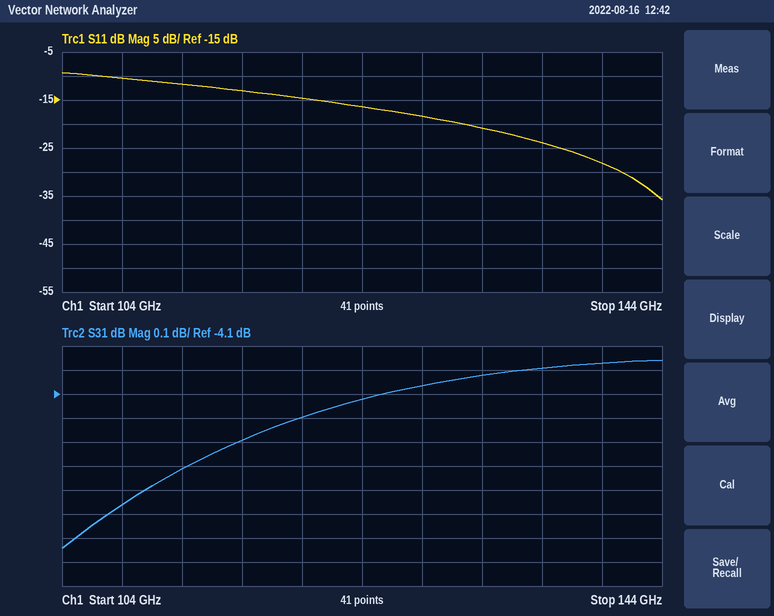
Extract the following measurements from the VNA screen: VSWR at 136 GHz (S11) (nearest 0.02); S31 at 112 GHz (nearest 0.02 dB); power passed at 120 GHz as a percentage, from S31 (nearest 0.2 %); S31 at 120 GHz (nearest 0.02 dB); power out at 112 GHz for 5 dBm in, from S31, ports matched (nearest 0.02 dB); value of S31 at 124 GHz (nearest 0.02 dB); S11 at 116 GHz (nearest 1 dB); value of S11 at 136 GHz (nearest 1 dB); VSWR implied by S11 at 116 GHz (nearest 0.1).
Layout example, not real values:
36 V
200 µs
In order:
1.14
-4.42 dB
38.0 %
-4.20 dB
0.58 dBm
-4.12 dB
-13 dB
-24 dB
1.6
